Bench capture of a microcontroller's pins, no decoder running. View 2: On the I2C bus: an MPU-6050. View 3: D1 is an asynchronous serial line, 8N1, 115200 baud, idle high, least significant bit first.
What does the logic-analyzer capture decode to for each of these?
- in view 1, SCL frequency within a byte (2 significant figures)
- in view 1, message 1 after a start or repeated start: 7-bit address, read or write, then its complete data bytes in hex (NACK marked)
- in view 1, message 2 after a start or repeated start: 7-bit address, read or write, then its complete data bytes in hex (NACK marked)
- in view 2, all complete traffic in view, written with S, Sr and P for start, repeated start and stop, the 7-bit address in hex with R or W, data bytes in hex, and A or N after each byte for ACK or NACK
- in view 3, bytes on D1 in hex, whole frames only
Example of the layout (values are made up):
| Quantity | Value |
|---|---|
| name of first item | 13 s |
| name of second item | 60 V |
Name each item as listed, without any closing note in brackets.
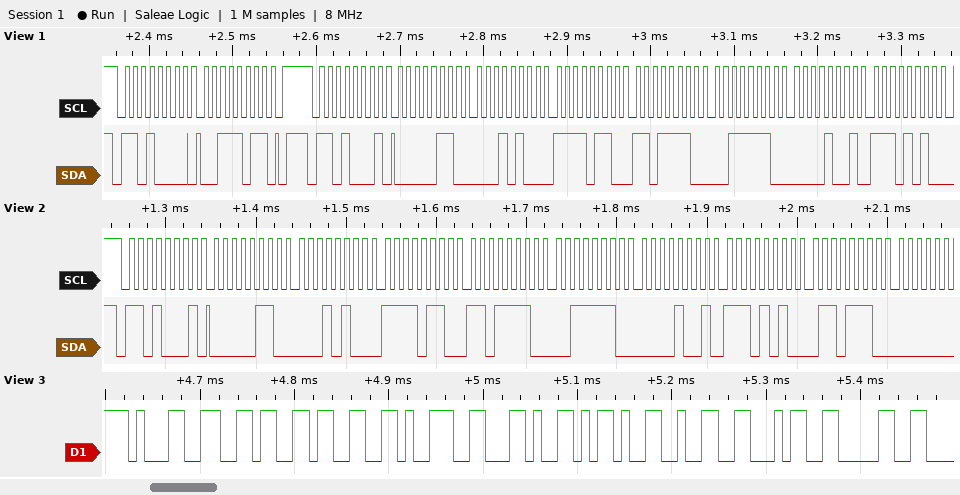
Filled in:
| Quantity | Value |
|---|---|
| in view 1, SCL frequency within a byte | 100 kHz |
| in view 1, message 1 after a start or repeated start: 7-bit address, read or write, then its complete data bytes in hex | 0x68 write: 3B |
| in view 1, message 2 after a start or repeated start: 7-bit address, read or write, then its complete data bytes in hex | 0x68 read: 06 14 F6 DE 3E 09 EA |
| in view 2, all complete traffic in view, written with S, Sr and P for start, repeated start and stop, the 7-bit address in hex with R or W, data bytes in hex, and A or N after each byte for ACK or NACK | S 68R A 06 A 14 A F6 A DE A 3E A 09 A EA A 6E A |
| in view 3, bytes on D1 in hex, whole frames only | 0x31 0x36 0x33 0x39 0x2C 0x2D 0x32 0x34 0x30 |
